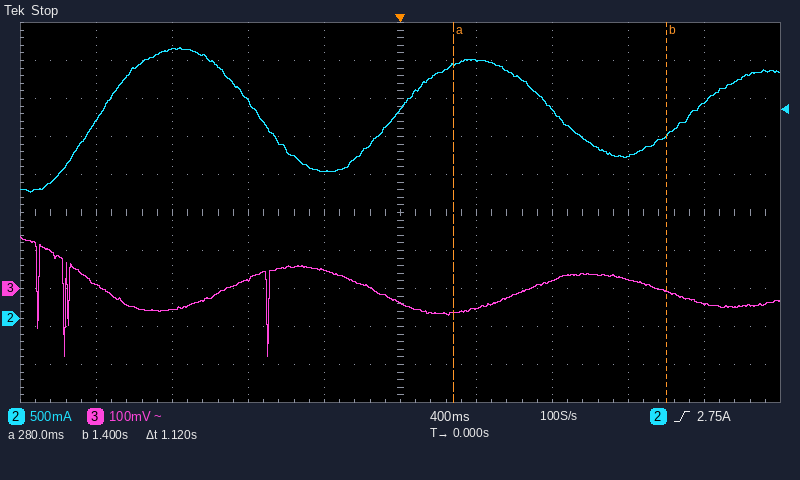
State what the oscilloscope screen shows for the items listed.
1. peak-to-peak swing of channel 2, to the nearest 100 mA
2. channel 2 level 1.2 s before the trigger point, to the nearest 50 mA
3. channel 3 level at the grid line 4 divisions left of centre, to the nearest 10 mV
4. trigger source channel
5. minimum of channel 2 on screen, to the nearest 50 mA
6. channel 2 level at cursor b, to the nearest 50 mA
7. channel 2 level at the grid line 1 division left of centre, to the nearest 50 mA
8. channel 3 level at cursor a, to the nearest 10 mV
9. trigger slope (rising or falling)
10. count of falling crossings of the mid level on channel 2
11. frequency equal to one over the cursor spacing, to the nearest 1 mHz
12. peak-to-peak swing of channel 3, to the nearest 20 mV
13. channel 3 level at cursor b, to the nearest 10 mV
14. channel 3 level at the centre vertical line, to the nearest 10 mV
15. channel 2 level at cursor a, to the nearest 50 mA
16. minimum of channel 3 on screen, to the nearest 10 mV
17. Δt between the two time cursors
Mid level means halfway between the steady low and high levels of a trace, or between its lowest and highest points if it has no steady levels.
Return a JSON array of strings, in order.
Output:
["1.90 A", "3.55 A", "10 mV", "channel 2", "1.65 A", "2.40 A", "1.95 A", "-60 mV", "rising", "2", "893 mHz", "320 mV", "-10 mV", "-40 mV", "3.35 A", "-180 mV", "1.12 s"]
